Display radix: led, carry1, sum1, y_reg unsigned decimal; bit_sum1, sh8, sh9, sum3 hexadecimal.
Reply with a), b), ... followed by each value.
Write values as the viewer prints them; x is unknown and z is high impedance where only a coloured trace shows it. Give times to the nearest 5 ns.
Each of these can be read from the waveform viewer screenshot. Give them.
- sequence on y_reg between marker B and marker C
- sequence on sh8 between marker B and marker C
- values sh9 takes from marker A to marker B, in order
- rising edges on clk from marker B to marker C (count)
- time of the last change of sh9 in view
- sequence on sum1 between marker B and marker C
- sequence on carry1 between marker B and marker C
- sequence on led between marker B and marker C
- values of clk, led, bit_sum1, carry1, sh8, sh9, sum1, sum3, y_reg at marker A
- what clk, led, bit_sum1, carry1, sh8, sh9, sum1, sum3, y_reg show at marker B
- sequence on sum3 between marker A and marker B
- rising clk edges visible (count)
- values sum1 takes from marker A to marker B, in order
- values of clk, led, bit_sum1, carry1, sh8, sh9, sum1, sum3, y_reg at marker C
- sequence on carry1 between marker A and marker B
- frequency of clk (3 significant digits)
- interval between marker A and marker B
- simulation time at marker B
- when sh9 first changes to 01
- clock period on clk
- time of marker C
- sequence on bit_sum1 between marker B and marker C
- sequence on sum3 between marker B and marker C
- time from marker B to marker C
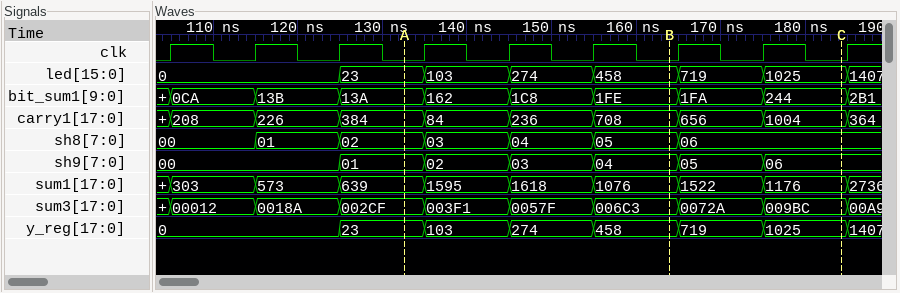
a) 458, 719, 1025
b) 05, 06
c) 01, 02, 03, 04
d) 2
e) 175 ns
f) 1076, 1522, 1176
g) 708, 656, 1004
h) 458, 719, 1025
i) clk=0, led=23, bit_sum1=13A, carry1=384, sh8=02, sh9=01, sum1=639, sum3=002CF, y_reg=23
j) clk=0, led=458, bit_sum1=1FE, carry1=708, sh8=05, sh9=04, sum1=1076, sum3=006C3, y_reg=458
k) 002CF, 003F1, 0057F, 006C3
l) 9
m) 639, 1595, 1618, 1076
n) clk=0, led=1025, bit_sum1=244, carry1=1004, sh8=06, sh9=06, sum1=1176, sum3=009BC, y_reg=1025
o) 384, 84, 236, 708
p) 100 MHz
q) 30 ns
r) 165 ns
s) 125 ns
t) 10 ns
u) 185 ns
v) 1FE, 1FA, 244
w) 006C3, 0072A, 009BC
x) 20 ns
